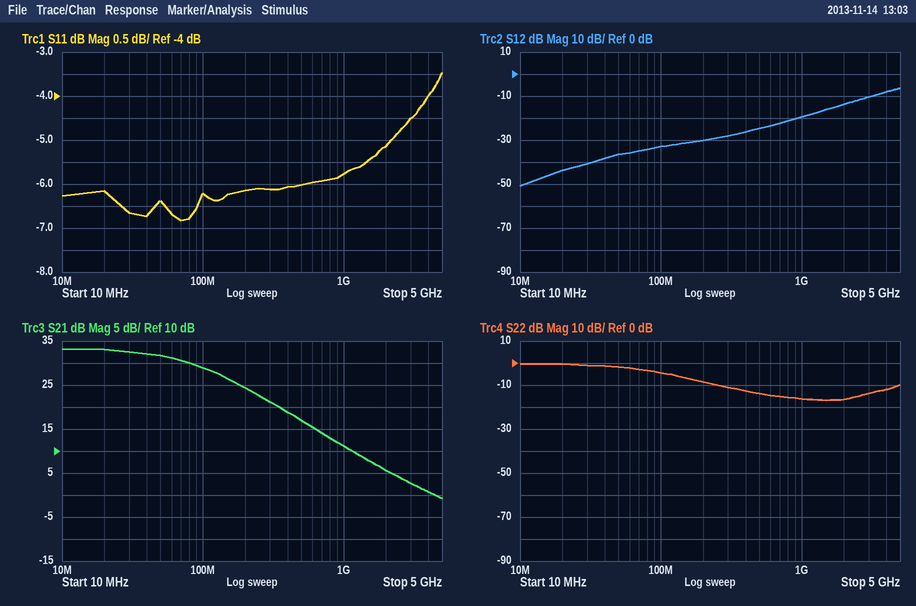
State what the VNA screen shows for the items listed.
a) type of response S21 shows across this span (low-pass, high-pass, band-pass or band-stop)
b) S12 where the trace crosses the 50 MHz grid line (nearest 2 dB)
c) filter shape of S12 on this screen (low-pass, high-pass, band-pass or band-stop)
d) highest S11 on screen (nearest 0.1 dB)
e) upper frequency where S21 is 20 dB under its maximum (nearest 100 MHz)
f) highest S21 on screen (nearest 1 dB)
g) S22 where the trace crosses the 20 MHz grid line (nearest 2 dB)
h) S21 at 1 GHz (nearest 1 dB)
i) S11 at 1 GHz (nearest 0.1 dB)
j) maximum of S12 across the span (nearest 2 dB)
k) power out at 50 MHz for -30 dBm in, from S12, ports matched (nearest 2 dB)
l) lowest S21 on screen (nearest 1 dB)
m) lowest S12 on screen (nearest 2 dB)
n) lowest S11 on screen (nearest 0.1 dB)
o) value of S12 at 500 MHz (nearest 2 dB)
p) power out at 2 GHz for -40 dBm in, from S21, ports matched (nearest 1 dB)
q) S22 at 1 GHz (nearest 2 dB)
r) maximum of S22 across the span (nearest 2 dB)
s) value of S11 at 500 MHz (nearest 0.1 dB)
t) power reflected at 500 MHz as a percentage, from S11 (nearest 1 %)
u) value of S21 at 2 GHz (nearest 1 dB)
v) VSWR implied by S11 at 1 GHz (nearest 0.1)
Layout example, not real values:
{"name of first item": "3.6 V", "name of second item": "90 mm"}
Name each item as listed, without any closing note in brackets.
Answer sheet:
{"type of response S21 shows across this span": "low-pass", "S12 where the trace crosses the 50 MHz grid line": "-36 dB", "filter shape of S12 on this screen": "high-pass", "highest S11 on screen": "-3.5 dB", "upper frequency where S21 is 20 dB under its maximum": "800 MHz", "highest S21 on screen": "33 dB", "S22 where the trace crosses the 20 MHz grid line": "0 dB", "S21 at 1 GHz": "11 dB", "S11 at 1 GHz": "-5.8 dB", "maximum of S12 across the span": "-6 dB", "power out at 50 MHz for -30 dBm in, from S12, ports matched": "-66 dBm", "lowest S21 on screen": "-1 dB", "lowest S12 on screen": "-50 dB", "lowest S11 on screen": "-6.8 dB", "value of S12 at 500 MHz": "-24 dB", "power out at 2 GHz for -40 dBm in, from S21, ports matched": "-34 dBm", "S22 at 1 GHz": "-16 dB", "maximum of S22 across the span": "0 dB", "value of S11 at 500 MHz": "-6.0 dB", "power reflected at 500 MHz as a percentage, from S11": "25 %", "value of S21 at 2 GHz": "6 dB", "VSWR implied by S11 at 1 GHz": "3.1"}
